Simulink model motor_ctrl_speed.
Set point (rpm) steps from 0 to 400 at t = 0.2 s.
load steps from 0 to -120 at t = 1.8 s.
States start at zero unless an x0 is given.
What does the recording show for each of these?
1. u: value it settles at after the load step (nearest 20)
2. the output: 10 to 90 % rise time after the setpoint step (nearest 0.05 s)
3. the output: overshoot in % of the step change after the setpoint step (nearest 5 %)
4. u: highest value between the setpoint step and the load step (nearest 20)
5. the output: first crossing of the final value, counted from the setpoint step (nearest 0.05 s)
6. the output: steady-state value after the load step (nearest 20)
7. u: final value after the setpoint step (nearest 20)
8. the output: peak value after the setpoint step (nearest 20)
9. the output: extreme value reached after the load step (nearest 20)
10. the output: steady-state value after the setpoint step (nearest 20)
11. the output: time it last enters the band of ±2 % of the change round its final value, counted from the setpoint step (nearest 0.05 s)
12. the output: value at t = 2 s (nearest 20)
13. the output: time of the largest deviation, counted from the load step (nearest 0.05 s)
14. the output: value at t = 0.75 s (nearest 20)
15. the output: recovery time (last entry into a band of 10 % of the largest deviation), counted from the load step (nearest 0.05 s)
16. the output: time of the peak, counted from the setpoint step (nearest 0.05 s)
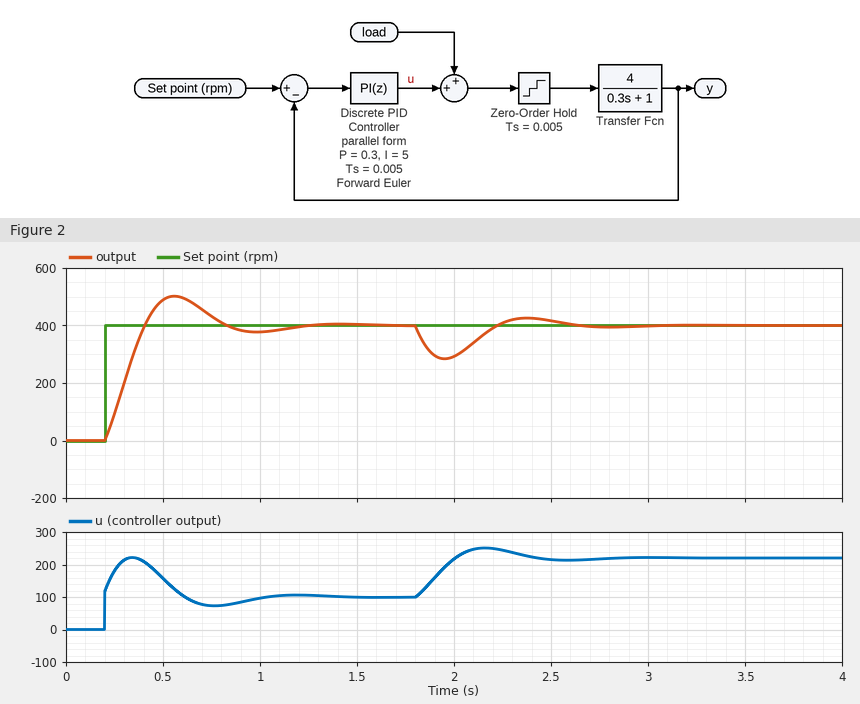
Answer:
220
0.15 s
25 %
220
0.20 s
400
100
500
280
400
0.95 s
300
0.15 s
440
0.75 s
0.35 s
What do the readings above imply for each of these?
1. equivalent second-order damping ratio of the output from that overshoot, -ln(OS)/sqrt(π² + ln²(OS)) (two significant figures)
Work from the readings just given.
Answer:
0.40
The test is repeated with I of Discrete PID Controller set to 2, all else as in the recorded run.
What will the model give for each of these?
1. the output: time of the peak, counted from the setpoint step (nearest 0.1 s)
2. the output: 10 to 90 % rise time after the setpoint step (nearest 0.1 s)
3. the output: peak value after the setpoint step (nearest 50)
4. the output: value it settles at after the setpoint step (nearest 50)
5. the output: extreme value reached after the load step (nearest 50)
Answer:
0.6 s
0.3 s
450
400
250
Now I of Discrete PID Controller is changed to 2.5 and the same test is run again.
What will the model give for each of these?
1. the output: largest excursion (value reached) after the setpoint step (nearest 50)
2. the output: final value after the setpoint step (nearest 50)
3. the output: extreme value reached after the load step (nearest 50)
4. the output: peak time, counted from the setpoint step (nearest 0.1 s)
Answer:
450
400
250
0.5 s
